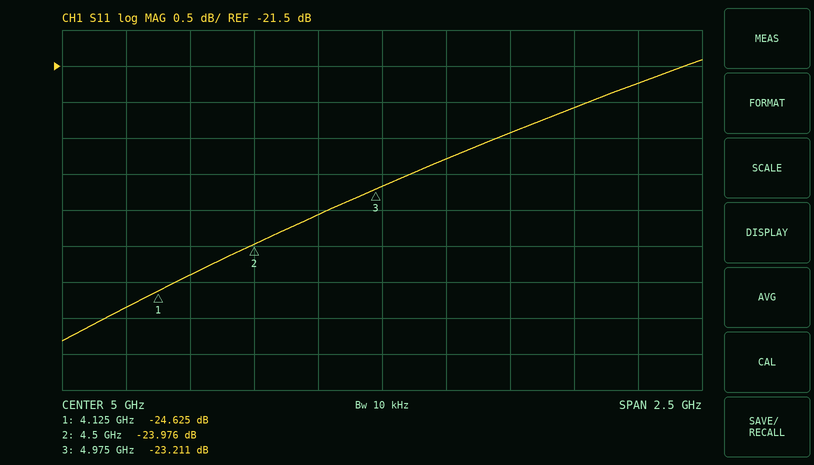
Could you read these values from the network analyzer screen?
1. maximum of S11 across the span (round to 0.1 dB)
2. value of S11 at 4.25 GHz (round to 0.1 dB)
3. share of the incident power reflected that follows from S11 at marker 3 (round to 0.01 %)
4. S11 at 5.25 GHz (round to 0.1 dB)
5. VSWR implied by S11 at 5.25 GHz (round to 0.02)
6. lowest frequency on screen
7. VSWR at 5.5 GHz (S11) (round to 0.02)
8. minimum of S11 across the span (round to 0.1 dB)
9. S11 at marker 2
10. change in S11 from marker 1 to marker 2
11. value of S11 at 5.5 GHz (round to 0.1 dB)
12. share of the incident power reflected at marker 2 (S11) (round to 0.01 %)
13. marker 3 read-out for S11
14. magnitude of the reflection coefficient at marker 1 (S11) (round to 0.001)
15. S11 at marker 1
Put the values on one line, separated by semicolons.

-21.4 dB; -24.4 dB; 0.48 %; -22.8 dB; 1.16; 3.75 GHz; 1.16; -25.3 dB; -23.976 dB; 0.649 dB; -22.4 dB; 0.40 %; -23.211 dB; 0.059; -24.625 dB
